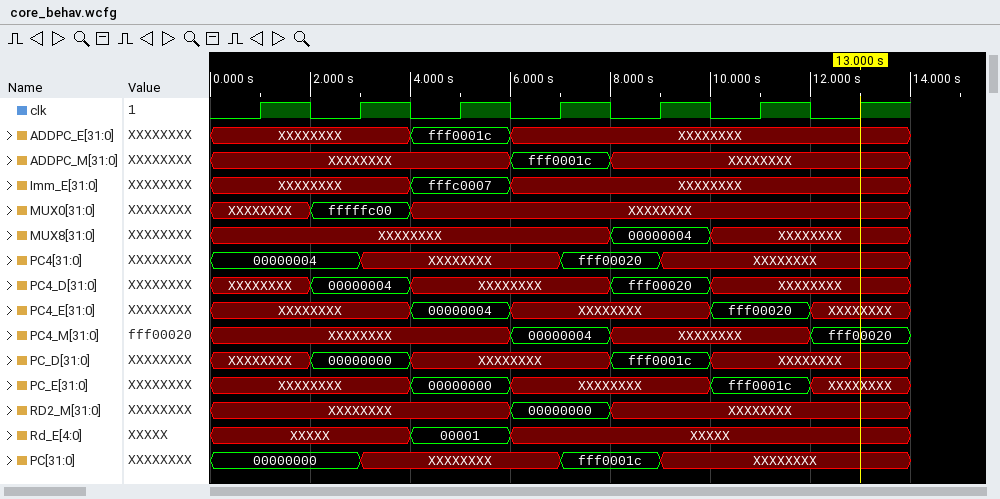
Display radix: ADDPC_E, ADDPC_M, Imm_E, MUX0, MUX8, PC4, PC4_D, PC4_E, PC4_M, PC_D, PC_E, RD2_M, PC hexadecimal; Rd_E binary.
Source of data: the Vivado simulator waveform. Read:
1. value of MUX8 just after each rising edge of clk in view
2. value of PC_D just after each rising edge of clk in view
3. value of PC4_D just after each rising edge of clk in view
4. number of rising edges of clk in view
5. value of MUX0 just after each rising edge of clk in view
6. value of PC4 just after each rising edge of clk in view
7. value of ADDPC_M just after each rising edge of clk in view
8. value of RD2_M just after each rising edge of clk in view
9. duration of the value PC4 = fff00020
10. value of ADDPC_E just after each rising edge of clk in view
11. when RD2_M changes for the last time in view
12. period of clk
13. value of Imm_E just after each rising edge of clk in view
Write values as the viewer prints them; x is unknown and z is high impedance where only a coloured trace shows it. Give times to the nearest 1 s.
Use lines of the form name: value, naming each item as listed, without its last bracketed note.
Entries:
value of MUX8 just after each rising edge of clk in view: XXXXXXXX, XXXXXXXX, XXXXXXXX, XXXXXXXX, 00000004, XXXXXXXX, XXXXXXXX
value of PC_D just after each rising edge of clk in view: XXXXXXXX, 00000000, XXXXXXXX, XXXXXXXX, fff0001c, XXXXXXXX, XXXXXXXX
value of PC4_D just after each rising edge of clk in view: XXXXXXXX, 00000004, XXXXXXXX, XXXXXXXX, fff00020, XXXXXXXX, XXXXXXXX
number of rising edges of clk in view: 7
value of MUX0 just after each rising edge of clk in view: XXXXXXXX, fffffc00, XXXXXXXX, XXXXXXXX, XXXXXXXX, XXXXXXXX, XXXXXXXX
value of PC4 just after each rising edge of clk in view: 00000004, XXXXXXXX, XXXXXXXX, fff00020, XXXXXXXX, XXXXXXXX, XXXXXXXX
value of ADDPC_M just after each rising edge of clk in view: XXXXXXXX, XXXXXXXX, XXXXXXXX, fff0001c, XXXXXXXX, XXXXXXXX, XXXXXXXX
value of RD2_M just after each rising edge of clk in view: XXXXXXXX, XXXXXXXX, XXXXXXXX, 00000000, XXXXXXXX, XXXXXXXX, XXXXXXXX
duration of the value PC4 = fff00020: 2 s
value of ADDPC_E just after each rising edge of clk in view: XXXXXXXX, XXXXXXXX, fff0001c, XXXXXXXX, XXXXXXXX, XXXXXXXX, XXXXXXXX
when RD2_M changes for the last time in view: 8 s
period of clk: 2 s
value of Imm_E just after each rising edge of clk in view: XXXXXXXX, XXXXXXXX, fffc0007, XXXXXXXX, XXXXXXXX, XXXXXXXX, XXXXXXXX
